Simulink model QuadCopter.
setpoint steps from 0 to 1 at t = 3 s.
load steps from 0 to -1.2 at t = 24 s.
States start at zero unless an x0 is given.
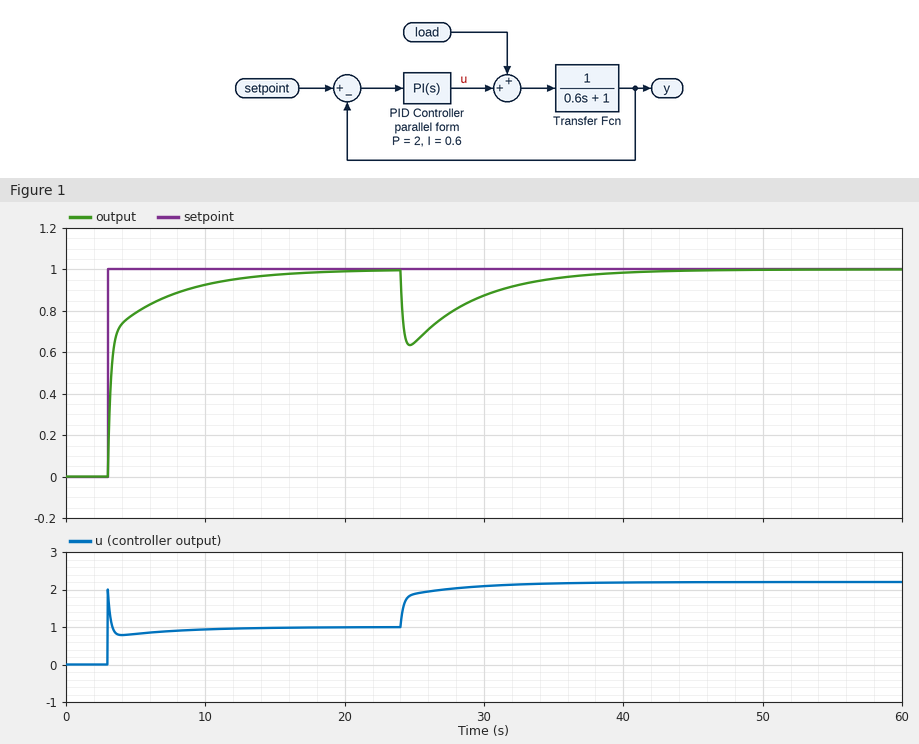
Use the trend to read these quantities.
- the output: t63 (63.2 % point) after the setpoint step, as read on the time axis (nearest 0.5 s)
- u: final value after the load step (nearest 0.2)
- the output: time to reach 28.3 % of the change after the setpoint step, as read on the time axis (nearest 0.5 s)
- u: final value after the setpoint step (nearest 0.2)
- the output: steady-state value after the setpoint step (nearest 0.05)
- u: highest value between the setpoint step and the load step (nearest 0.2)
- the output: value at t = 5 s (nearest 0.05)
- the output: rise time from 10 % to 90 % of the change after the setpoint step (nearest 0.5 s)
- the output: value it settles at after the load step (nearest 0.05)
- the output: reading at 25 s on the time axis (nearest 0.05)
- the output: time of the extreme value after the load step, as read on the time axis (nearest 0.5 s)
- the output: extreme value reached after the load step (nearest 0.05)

3.5 s
2.2
3.0 s
1.0
1.00
2.0
0.80
5.5 s
1.00
0.65
24.5 s
0.65
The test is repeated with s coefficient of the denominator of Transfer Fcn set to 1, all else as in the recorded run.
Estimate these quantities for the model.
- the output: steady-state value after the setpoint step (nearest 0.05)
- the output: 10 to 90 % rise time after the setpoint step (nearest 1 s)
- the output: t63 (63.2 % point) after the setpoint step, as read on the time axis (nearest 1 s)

1.00
5 s
4 s
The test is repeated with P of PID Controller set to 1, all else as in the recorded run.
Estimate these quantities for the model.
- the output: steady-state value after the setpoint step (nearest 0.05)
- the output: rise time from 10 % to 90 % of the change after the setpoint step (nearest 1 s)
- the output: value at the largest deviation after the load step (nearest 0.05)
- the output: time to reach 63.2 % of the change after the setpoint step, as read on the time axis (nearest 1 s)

1.00
5 s
0.50
4 s
